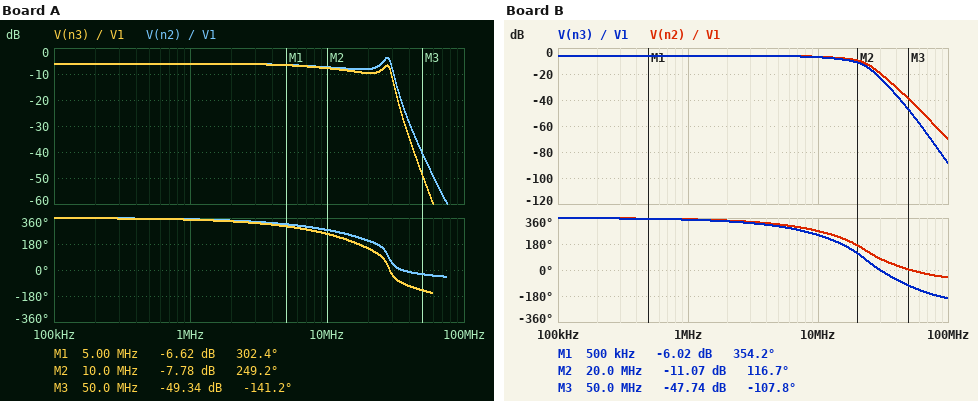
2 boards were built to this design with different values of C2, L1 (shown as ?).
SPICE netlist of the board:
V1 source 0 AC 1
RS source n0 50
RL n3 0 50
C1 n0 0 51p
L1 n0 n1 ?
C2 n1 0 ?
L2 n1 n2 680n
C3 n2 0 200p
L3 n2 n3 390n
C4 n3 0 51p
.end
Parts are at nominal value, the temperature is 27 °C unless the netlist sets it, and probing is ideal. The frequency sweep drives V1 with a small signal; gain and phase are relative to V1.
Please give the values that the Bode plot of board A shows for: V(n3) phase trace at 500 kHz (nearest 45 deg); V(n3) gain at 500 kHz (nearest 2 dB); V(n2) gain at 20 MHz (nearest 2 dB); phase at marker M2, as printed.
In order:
360 deg
-6 dB
-8 dB
249.2 deg
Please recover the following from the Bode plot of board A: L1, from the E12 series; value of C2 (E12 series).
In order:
1.2 µH
100 pF
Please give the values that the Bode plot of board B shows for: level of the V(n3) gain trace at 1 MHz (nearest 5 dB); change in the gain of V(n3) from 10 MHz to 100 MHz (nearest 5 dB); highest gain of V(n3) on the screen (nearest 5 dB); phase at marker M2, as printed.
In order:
-5 dB
-80 dB
-5 dB
116.7 deg
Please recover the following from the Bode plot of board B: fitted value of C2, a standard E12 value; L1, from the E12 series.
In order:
470 pF
220 nH
